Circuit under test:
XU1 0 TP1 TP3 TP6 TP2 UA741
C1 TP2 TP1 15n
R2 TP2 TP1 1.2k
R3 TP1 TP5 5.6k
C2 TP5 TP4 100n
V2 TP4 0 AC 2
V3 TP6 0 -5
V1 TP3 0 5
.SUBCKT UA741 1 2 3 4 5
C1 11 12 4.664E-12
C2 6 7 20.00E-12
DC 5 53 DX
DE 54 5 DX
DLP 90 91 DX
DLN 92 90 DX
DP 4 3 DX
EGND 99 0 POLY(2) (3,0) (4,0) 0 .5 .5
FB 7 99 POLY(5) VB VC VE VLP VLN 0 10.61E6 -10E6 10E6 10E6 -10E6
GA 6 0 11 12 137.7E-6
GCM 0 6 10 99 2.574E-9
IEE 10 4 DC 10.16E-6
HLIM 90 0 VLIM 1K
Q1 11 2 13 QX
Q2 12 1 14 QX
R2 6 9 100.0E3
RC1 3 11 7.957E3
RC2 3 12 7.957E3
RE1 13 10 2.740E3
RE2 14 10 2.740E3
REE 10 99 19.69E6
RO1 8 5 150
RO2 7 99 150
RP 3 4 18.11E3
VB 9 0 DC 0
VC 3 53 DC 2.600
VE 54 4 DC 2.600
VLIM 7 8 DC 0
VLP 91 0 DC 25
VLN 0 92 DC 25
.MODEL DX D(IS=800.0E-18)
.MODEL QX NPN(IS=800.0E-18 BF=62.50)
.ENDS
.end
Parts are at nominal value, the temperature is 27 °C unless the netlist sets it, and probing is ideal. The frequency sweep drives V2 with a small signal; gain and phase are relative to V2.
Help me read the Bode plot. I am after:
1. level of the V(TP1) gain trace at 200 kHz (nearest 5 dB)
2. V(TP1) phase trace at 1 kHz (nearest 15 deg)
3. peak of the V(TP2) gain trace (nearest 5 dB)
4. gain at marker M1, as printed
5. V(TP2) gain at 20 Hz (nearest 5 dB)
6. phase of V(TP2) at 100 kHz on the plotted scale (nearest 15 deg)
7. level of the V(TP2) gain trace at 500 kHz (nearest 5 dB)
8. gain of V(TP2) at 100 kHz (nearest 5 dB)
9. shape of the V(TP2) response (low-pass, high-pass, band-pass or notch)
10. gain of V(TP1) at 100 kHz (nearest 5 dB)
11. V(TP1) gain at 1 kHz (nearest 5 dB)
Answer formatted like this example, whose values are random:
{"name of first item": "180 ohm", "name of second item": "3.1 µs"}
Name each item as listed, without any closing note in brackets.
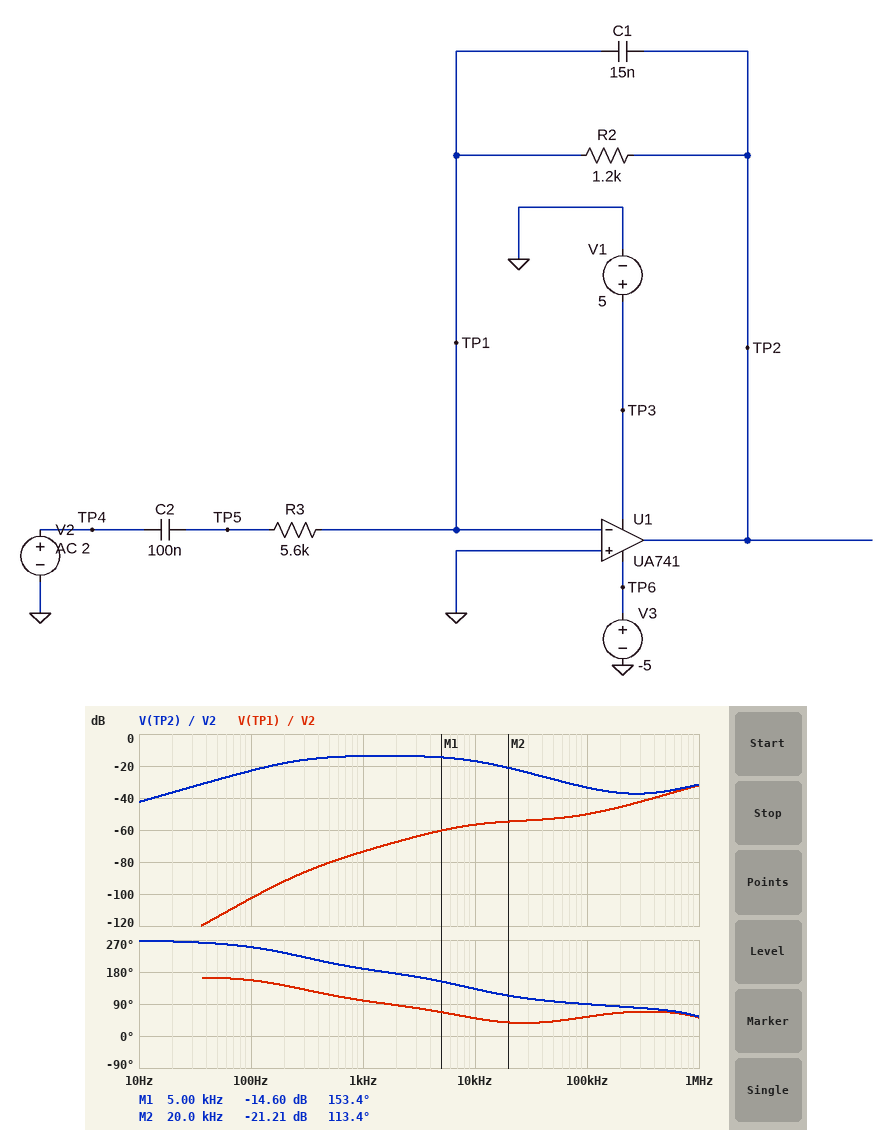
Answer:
{"level of the V(TP1) gain trace at 200 kHz": "-45 dB", "V(TP1) phase trace at 1 kHz": "105 deg", "peak of the V(TP2) gain trace": "-15 dB", "gain at marker M1, as printed": "-14.60 dB", "V(TP2) gain at 20 Hz": "-35 dB", "phase of V(TP2) at 100 kHz on the plotted scale": "90 deg", "level of the V(TP2) gain trace at 500 kHz": "-35 dB", "gain of V(TP2) at 100 kHz": "-35 dB", "shape of the V(TP2) response": "band-pass", "gain of V(TP1) at 100 kHz": "-50 dB", "V(TP1) gain at 1 kHz": "-75 dB"}
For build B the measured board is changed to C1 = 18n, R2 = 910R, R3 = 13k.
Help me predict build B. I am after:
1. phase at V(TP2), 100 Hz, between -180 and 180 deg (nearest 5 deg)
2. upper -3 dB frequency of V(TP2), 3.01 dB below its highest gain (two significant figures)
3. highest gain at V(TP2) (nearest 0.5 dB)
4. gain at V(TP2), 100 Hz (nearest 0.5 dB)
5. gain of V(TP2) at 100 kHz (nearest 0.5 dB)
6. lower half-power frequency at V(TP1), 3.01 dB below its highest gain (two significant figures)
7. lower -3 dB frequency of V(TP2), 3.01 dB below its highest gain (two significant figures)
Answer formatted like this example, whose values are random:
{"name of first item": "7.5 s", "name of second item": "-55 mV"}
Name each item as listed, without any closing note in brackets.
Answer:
{"phase at V(TP2), 100 Hz, between -180 and 180 deg": "-130 deg", "upper -3 dB frequency of V(TP2), 3.01 dB below its highest gain": "10 kHz", "highest gain at V(TP2)": "-23.0 dB", "gain at V(TP2), 100 Hz": "-27.0 dB", "gain of V(TP2) at 100 kHz": "-42.0 dB", "lower half-power frequency at V(TP1), 3.01 dB below its highest gain": "950 kHz", "lower -3 dB frequency of V(TP2), 3.01 dB below its highest gain": "120 Hz"}
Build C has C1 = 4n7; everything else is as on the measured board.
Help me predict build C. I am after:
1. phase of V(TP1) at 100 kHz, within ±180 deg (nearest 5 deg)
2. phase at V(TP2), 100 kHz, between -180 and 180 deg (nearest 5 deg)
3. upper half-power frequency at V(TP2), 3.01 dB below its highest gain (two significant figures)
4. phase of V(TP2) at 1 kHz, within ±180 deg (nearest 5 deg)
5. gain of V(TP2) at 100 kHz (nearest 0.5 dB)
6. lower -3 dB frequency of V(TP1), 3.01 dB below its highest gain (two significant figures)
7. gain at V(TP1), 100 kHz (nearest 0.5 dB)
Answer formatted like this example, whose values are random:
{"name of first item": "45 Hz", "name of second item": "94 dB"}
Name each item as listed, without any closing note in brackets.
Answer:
{"phase of V(TP1) at 100 kHz, within ±180 deg": "35 deg", "phase at V(TP2), 100 kHz, between -180 and 180 deg": "100 deg", "upper half-power frequency at V(TP2), 3.01 dB below its highest gain": "29 kHz", "phase of V(TP2) at 1 kHz, within ±180 deg": "-165 deg", "gain of V(TP2) at 100 kHz": "-24.5 dB", "lower -3 dB frequency of V(TP1), 3.01 dB below its highest gain": "920 kHz", "gain at V(TP1), 100 kHz": "-44.0 dB"}
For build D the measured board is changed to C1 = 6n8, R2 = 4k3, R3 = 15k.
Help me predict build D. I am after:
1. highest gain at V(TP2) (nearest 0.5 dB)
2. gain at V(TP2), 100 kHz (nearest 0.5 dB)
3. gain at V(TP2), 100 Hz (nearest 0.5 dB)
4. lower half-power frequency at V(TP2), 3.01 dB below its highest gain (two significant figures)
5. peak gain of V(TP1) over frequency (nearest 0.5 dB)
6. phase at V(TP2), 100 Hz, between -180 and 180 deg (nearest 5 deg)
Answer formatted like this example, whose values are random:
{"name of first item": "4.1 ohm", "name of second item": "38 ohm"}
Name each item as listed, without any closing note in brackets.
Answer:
{"highest gain at V(TP2)": "-11.0 dB", "gain at V(TP2), 100 kHz": "-35.5 dB", "gain at V(TP2), 100 Hz": "-14.0 dB", "lower half-power frequency at V(TP2), 3.01 dB below its highest gain": "100 Hz", "peak gain of V(TP1) over frequency": "-38.0 dB", "phase at V(TP2), 100 Hz, between -180 and 180 deg": "-135 deg"}
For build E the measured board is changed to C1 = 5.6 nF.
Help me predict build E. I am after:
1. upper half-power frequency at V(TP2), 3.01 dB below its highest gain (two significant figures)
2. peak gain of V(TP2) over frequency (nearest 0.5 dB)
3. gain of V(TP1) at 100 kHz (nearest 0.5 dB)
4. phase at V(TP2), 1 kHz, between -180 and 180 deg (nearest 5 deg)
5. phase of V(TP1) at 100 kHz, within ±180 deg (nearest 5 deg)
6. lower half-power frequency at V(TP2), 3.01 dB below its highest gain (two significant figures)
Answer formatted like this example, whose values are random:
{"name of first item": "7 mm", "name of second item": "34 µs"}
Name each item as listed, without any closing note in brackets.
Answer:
{"upper half-power frequency at V(TP2), 3.01 dB below its highest gain": "24 kHz", "peak gain of V(TP2) over frequency": "-13.5 dB", "gain of V(TP1) at 100 kHz": "-45.0 dB", "phase at V(TP2), 1 kHz, between -180 and 180 deg": "-165 deg", "phase of V(TP1) at 100 kHz, within ±180 deg": "35 deg", "lower half-power frequency at V(TP2), 3.01 dB below its highest gain": "280 Hz"}
